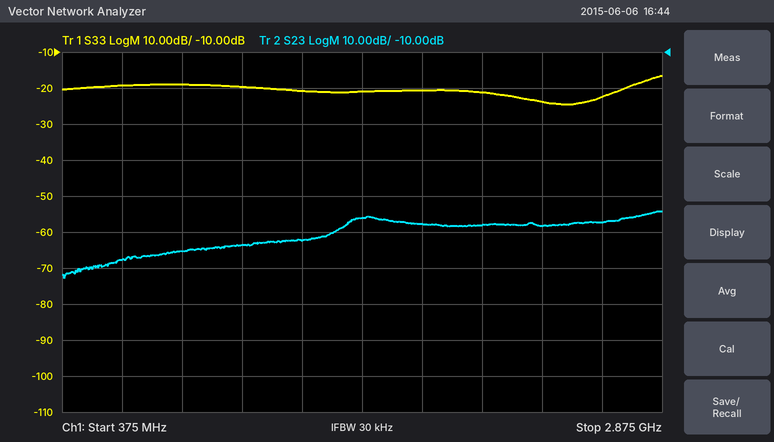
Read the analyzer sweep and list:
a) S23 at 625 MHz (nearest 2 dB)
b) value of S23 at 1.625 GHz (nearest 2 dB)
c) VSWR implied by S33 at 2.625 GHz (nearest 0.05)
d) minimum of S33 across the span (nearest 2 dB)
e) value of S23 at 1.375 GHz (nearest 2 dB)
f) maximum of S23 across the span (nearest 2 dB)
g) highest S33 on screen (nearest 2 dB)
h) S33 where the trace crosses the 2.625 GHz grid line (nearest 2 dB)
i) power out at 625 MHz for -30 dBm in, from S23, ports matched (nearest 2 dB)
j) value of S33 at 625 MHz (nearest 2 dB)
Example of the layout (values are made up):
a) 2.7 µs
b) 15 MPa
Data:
a) -68 dB
b) -56 dB
c) 1.15
d) -24 dB
e) -62 dB
f) -54 dB
g) -16 dB
h) -22 dB
i) -98 dBm
j) -20 dB
